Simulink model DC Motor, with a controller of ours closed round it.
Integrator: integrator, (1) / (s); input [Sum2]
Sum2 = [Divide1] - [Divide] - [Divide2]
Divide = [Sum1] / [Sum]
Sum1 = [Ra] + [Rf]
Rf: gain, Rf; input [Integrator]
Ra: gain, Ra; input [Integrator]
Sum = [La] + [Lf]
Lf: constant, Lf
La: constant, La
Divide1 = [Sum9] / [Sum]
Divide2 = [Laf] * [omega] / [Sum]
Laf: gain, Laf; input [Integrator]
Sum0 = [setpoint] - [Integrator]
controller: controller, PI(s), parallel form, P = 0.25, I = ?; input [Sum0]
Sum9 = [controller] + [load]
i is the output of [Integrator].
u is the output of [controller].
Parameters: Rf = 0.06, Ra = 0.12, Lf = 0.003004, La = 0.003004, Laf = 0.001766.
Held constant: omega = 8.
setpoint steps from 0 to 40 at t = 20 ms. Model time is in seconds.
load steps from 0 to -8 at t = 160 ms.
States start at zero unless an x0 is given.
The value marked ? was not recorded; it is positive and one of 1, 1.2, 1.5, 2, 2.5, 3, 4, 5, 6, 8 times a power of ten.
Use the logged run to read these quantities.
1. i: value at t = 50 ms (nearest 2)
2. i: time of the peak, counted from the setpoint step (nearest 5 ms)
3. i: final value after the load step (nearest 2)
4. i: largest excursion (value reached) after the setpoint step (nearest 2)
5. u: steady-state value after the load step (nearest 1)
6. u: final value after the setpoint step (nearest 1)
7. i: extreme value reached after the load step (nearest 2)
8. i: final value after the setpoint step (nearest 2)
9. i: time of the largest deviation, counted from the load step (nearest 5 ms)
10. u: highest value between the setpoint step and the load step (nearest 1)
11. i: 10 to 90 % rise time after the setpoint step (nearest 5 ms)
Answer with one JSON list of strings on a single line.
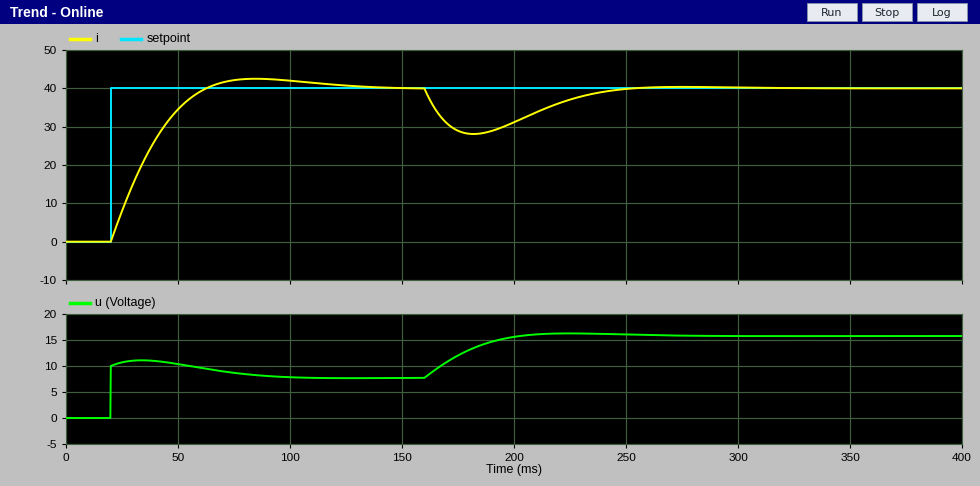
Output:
["34", "65 ms", "40", "42", "16", "8", "28", "40", "20 ms", "11", "30 ms"]
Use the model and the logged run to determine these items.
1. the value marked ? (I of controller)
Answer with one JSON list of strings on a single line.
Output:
["15"]
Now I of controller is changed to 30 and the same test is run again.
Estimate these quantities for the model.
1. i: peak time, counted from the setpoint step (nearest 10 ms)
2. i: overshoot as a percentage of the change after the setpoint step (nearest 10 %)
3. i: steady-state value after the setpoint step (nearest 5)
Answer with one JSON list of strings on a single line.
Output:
["40 ms", "20 %", "40"]
